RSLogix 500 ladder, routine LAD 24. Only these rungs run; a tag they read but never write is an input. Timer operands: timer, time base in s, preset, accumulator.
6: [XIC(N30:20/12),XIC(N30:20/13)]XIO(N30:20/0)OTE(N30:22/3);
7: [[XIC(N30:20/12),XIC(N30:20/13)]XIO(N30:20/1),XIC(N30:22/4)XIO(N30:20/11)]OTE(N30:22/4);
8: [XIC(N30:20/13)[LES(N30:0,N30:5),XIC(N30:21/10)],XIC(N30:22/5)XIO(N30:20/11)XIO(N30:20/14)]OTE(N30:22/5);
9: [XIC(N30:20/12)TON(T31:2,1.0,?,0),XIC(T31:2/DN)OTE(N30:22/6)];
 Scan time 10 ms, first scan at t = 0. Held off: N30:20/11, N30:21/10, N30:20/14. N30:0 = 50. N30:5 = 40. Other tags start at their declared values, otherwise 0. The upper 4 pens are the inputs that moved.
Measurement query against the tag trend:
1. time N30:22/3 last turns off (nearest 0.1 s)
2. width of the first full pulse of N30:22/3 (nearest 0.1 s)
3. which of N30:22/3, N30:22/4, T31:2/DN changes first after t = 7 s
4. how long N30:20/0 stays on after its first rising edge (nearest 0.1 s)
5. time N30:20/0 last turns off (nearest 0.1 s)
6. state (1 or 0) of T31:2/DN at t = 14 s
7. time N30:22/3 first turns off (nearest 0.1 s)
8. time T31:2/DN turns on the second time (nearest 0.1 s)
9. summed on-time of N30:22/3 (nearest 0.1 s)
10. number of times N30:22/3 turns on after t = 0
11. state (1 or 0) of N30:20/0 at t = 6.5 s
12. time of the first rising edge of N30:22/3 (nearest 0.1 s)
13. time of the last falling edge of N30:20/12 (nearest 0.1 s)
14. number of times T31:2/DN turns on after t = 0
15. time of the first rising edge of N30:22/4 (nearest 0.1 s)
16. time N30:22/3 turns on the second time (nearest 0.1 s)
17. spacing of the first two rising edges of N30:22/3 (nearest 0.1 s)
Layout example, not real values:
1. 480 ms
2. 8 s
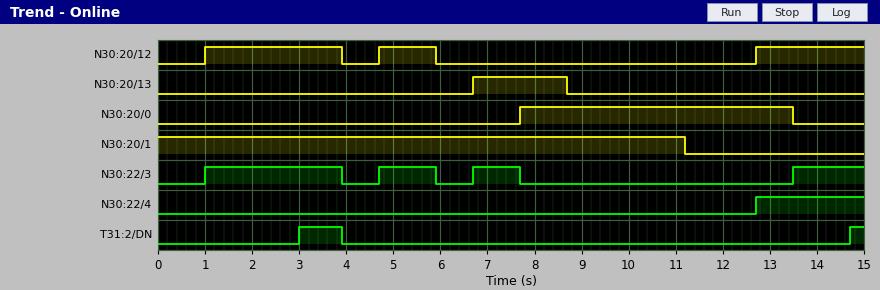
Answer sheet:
1. 7.7 s
2. 2.9 s
3. N30:22/3
4. 5.8 s
5. 13.5 s
6. 0
7. 3.9 s
8. 14.7 s
9. 6.6 s
10. 4
11. 0
12. 1.0 s
13. 5.9 s
14. 2
15. 12.7 s
16. 4.7 s
17. 3.7 s
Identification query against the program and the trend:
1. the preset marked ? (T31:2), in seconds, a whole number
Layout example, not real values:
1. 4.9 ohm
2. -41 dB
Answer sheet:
1. 2 s
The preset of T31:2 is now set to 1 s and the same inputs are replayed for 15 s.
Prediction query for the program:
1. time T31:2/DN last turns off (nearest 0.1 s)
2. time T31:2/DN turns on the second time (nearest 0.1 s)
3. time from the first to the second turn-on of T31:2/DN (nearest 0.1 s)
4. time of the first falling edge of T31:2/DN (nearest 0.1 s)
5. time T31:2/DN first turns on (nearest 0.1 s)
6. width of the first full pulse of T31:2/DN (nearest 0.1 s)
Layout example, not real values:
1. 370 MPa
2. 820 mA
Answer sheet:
1. 5.9 s
2. 5.7 s
3. 3.7 s
4. 3.9 s
5. 2.0 s
6. 1.9 s
